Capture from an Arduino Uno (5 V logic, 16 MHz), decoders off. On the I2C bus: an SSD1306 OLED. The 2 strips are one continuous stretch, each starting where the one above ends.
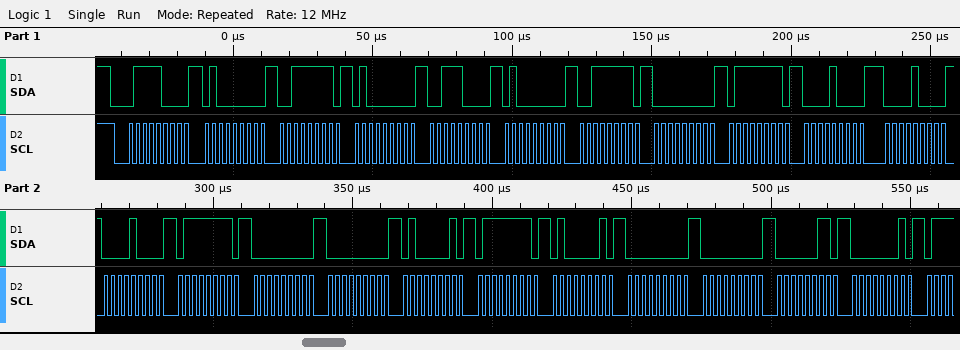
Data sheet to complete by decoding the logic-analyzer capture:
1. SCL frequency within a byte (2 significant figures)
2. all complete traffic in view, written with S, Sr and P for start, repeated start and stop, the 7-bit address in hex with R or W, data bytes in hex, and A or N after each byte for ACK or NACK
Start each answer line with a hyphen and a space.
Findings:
- 400 kHz
- S 3CW A 40 A 3F A 40 A 38 A 40 A 3F A 00 A 7F A 08 A 08 A 08 A 7F A 00 A 00 A 41 A 7F A 41 A 00 A 00 A 03 A 01 A
